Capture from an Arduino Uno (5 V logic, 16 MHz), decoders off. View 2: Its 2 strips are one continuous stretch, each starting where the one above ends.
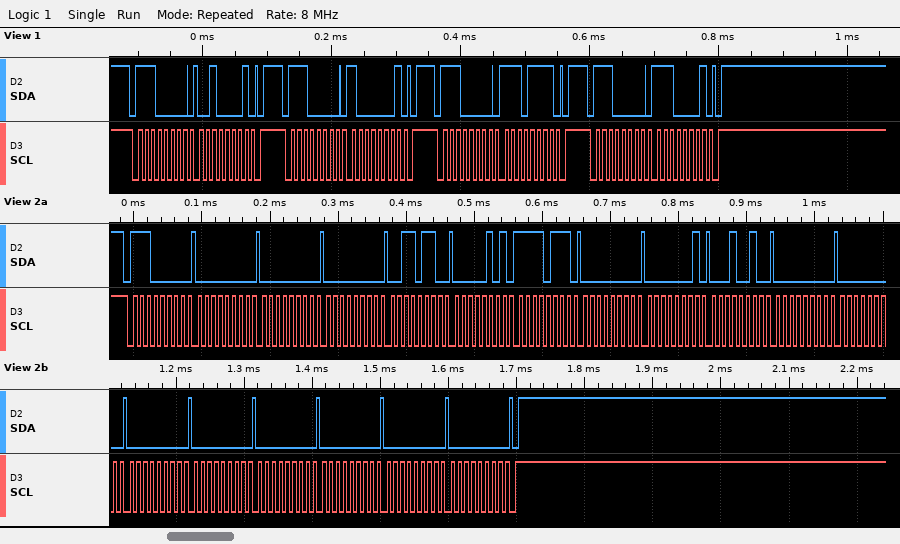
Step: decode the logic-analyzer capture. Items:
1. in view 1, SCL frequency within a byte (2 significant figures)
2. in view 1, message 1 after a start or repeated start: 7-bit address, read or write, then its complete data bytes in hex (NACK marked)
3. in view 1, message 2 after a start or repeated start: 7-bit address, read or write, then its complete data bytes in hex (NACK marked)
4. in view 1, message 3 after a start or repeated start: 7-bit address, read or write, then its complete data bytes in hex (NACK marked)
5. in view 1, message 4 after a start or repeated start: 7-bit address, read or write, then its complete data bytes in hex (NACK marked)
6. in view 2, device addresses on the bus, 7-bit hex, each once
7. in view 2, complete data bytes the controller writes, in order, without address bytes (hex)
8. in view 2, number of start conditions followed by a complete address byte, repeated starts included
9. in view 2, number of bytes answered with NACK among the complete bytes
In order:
100 kHz
0x70 write: 21
0x70 write: 81
0x70 write: EF
0x70 write: E1
0x70
00 00 00 36 05 F7 00 01 12 00 00 00 00 00 00 00 00
1
0
